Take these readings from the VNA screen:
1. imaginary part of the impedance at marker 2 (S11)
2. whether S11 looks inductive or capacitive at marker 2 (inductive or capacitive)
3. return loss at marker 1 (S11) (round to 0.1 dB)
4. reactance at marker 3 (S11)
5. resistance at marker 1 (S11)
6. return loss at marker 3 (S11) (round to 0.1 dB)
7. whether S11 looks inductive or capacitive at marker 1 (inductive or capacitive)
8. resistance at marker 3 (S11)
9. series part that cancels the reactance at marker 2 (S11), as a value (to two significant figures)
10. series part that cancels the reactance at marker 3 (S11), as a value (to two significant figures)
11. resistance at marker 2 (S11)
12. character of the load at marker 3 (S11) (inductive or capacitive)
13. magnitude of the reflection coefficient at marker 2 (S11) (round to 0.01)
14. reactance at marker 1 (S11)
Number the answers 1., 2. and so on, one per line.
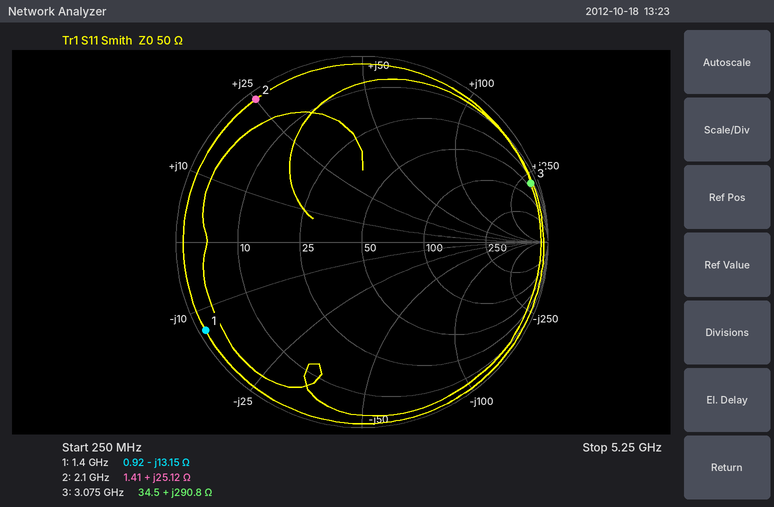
1. +25.12 Ω
2. inductive
3. 0.3 dB
4. +290.8 Ω
5. 0.92 Ω
6. 0.3 dB
7. capacitive
8. 34.5 Ω
9. 3.0 pF
10. 180 fF
11. 1.41 Ω
12. inductive
13. 0.96
14. -13.15 Ω
